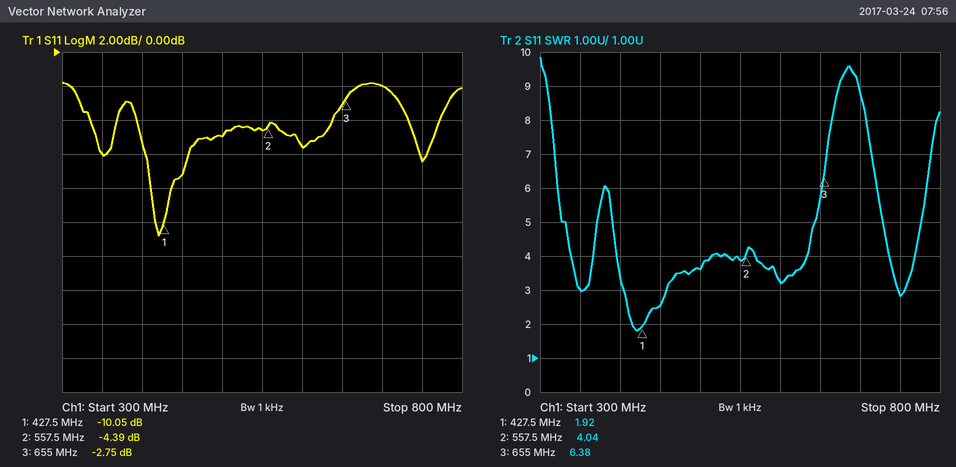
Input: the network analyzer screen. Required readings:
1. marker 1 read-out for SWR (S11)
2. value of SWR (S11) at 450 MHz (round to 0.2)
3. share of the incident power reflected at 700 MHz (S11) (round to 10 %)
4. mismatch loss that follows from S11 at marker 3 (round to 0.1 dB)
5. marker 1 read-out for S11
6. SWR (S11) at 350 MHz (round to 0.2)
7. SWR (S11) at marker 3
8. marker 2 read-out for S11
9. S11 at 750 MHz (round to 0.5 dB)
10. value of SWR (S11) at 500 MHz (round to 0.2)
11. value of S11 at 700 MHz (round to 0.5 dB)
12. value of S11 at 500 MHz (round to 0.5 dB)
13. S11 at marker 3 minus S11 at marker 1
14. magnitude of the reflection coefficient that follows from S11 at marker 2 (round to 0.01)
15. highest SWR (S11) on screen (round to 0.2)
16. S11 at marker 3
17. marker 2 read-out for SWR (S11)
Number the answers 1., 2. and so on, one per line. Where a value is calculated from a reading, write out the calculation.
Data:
1. 1.92
2. 2.6
3. 10^(-2/10) ≈ 63.1 %, so 60 % to the nearest 10 %
4. −10 log10(1 − 10^(-2.75/10)) ≈ 3.3 dB
5. -10.05 dB
6. 3.0
7. 6.38
8. -4.39 dB
9. -6.5 dB
10. 3.6
11. -2.0 dB
12. -5.0 dB
13. -2.75 − (-10.05) = 7.30 dB
14. 10^(-4.39/20) ≈ 0.60
15. 9.8
16. -2.75 dB
17. 4.04
